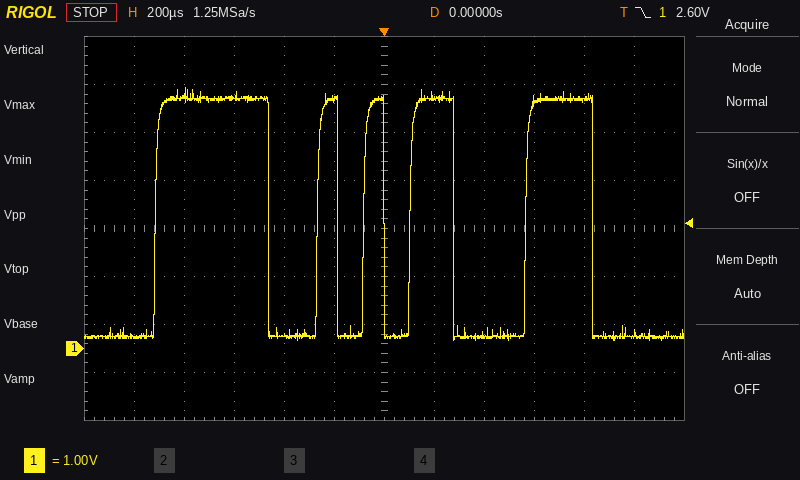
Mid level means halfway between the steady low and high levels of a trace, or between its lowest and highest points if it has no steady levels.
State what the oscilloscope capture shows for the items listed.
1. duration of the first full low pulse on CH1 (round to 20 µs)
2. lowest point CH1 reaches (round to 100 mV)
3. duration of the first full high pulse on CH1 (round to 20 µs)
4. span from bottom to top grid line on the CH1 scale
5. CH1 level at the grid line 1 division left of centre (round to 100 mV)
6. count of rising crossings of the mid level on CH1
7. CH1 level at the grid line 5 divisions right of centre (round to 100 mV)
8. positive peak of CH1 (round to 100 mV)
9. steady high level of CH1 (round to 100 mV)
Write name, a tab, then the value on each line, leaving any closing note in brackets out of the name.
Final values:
duration of the first full low pulse on CH1	200 µs
lowest point CH1 reaches	200 mV
duration of the first full high pulse on CH1	460 µs
span from bottom to top grid line on the CH1 scale	8 V
CH1 level at the grid line 1 division left of centre	5.2 V
count of rising crossings of the mid level on CH1	5
CH1 level at the grid line 5 divisions right of centre	300 mV
positive peak of CH1	5.4 V
steady high level of CH1	5.2 V
